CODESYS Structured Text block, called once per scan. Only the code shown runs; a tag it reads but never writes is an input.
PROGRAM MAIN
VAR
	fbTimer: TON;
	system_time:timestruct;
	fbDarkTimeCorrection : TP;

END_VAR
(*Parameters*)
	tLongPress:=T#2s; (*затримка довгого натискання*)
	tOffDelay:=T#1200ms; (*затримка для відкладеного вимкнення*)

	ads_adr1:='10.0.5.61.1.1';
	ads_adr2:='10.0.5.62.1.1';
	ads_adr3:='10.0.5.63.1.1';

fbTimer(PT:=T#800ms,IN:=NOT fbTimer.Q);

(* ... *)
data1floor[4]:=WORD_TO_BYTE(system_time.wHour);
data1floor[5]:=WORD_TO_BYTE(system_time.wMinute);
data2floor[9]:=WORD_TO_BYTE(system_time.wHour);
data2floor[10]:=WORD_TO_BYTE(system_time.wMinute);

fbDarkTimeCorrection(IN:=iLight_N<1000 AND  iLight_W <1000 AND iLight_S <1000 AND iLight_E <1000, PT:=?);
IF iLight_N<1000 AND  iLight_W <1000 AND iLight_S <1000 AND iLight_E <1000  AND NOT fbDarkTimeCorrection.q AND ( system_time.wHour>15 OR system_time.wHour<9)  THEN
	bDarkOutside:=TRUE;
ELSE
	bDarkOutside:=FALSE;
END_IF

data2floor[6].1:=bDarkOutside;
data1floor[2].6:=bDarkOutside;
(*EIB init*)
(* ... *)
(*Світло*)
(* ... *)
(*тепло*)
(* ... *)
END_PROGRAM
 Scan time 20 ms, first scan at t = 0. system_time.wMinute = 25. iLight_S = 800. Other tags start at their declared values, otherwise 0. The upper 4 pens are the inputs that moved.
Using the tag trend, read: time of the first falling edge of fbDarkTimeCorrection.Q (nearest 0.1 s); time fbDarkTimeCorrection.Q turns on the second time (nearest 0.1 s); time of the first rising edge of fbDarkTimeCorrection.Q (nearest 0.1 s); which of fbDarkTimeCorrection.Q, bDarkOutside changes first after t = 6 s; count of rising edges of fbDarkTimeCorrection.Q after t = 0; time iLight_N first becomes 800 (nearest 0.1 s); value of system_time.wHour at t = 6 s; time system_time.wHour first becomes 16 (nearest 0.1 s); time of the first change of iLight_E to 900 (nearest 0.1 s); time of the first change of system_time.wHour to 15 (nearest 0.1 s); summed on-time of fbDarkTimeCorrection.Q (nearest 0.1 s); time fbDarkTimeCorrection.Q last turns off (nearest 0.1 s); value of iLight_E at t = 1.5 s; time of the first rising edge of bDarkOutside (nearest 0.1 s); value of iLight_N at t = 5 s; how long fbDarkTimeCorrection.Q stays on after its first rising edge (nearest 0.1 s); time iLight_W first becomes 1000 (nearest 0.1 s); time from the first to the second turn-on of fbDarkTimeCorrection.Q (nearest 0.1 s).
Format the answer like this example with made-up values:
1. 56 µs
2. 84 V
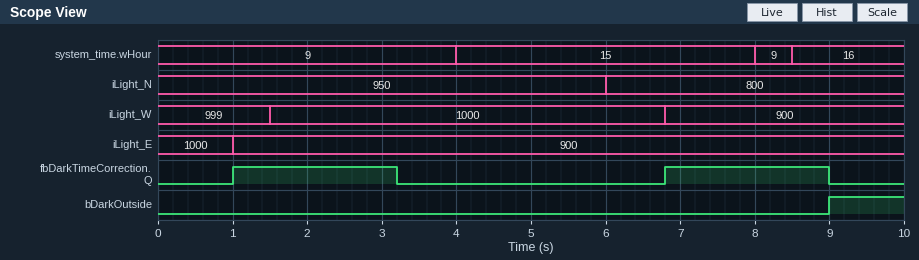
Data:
1. 3.2 s
2. 6.8 s
3. 1.0 s
4. fbDarkTimeCorrection.Q
5. 2
6. 6.0 s
7. 15
8. 8.5 s
9. 1.0 s
10. 4.0 s
11. 4.4 s
12. 9.0 s
13. 900
14. 9.0 s
15. 950
16. 2.2 s
17. 1.5 s
18. 5.8 s
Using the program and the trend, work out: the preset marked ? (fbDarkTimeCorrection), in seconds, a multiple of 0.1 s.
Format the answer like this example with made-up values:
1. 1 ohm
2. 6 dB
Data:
1. 2.2 s
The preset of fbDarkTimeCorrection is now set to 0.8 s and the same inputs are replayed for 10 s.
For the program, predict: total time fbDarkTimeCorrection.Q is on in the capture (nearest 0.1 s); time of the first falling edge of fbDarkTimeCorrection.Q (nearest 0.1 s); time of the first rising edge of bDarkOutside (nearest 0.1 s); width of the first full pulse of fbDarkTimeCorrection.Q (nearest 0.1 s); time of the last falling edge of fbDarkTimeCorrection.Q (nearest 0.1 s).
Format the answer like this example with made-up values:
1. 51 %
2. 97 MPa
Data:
1. 1.6 s
2. 1.8 s
3. 8.5 s
4. 0.8 s
5. 7.6 s
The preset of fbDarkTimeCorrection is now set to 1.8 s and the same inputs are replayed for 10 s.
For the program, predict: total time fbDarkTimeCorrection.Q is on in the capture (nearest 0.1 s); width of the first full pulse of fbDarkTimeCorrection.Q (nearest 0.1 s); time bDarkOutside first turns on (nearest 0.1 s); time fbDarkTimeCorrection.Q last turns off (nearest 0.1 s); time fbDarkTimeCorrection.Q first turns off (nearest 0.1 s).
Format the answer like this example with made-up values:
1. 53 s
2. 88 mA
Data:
1. 3.6 s
2. 1.8 s
3. 8.6 s
4. 8.6 s
5. 2.8 s
